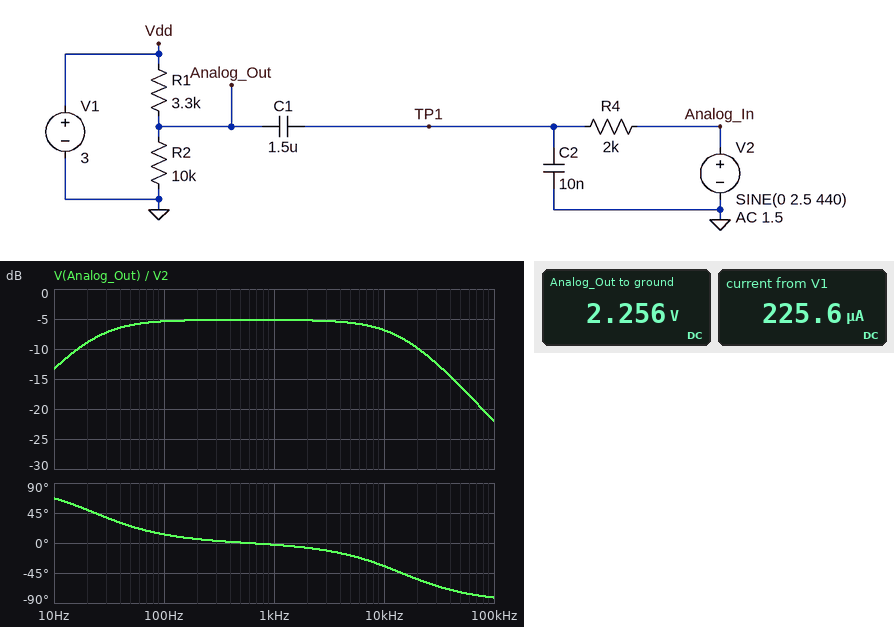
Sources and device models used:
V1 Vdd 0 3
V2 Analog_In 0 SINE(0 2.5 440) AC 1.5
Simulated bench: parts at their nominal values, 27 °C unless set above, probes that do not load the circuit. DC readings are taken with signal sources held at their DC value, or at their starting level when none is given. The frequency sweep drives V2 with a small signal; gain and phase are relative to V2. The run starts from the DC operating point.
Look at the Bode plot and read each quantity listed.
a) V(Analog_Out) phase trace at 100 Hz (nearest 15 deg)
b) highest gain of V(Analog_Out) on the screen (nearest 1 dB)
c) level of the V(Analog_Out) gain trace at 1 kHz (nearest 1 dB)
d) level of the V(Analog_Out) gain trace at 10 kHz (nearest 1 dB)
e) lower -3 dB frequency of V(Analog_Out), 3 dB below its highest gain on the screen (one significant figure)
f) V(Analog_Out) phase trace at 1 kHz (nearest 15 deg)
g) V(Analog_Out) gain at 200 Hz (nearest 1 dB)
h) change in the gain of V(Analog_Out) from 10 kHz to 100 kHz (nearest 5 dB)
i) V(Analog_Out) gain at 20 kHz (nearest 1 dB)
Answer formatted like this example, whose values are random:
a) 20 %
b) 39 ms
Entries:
a) 15 deg
b) -5 dB
c) -5 dB
d) -7 dB
e) 20 Hz
f) 0 deg
g) -5 dB
h) -15 dB
i) -10 dB
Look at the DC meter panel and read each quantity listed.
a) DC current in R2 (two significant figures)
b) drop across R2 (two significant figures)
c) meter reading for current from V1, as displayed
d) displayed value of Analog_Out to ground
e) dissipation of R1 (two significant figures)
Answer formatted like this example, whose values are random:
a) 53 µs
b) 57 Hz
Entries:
a) 230 µA
b) 2.3 V
c) 225.6 µA
d) 2.256 V
e) 170 µW
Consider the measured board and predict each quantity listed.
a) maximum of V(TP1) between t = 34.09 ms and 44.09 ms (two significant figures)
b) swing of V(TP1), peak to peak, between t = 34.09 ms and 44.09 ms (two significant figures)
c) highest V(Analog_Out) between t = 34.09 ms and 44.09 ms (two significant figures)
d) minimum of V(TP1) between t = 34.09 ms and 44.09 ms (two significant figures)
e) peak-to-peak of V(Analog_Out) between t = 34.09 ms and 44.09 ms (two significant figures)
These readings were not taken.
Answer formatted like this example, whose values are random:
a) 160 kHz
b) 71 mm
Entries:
a) 1.4 V
b) 2.8 V
c) 3.6 V
d) -1.4 V
e) 2.8 V
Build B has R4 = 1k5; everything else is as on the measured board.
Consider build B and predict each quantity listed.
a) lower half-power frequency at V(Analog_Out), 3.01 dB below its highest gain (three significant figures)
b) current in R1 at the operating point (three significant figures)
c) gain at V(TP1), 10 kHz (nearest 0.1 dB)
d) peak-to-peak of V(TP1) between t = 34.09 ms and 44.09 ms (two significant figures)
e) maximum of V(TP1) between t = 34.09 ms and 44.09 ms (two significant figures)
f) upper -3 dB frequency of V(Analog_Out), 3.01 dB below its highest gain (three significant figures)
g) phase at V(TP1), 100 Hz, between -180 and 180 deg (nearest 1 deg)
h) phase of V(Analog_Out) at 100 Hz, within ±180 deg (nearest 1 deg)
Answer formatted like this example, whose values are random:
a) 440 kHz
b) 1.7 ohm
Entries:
a) 26.5 Hz
b) 226 µA
c) -5.4 dB
d) 3.1 V
e) 1.6 V
f) 17.1 kHz
g) -9 deg
h) 15 deg
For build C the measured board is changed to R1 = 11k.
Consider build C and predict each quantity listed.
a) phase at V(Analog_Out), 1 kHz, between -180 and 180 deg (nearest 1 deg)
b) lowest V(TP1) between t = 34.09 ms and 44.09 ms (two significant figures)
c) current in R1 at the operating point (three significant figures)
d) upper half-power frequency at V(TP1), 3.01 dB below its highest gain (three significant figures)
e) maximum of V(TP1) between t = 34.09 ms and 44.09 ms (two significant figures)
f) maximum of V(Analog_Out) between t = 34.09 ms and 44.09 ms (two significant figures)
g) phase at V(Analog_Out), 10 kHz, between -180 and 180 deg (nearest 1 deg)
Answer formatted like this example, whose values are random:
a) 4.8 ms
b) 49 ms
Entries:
a) -4 deg
b) -1.8 V
c) 143 µA
d) 2.37 kHz
e) 1.8 V
f) 3.2 V
g) -42 deg
